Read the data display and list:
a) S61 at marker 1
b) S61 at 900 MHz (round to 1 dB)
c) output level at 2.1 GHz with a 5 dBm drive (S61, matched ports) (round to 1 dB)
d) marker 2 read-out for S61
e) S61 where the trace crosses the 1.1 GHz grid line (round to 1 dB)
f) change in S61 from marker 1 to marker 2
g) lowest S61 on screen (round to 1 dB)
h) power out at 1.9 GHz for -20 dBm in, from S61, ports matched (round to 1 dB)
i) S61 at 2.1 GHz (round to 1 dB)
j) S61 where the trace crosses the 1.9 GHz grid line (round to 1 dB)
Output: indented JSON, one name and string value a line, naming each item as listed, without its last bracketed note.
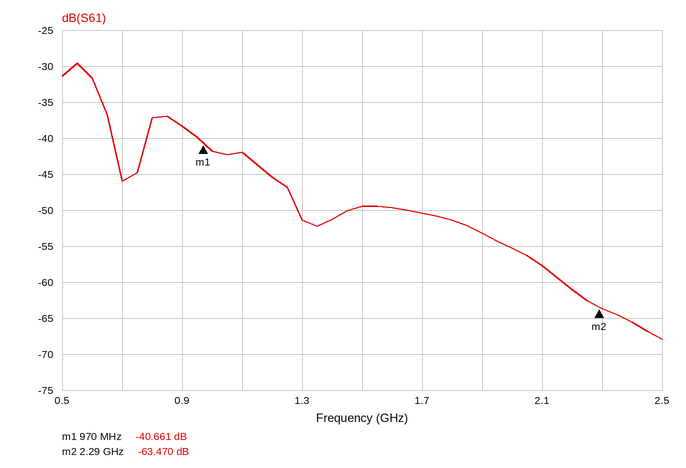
{
  "S61 at marker 1": "-40.661 dB",
  "S61 at 900 MHz": "-38 dB",
  "output level at 2.1 GHz with a 5 dBm drive (S61, matched ports)": "-53 dBm",
  "marker 2 read-out for S61": "-63.470 dB",
  "S61 where the trace crosses the 1.1 GHz grid line": "-42 dB",
  "change in S61 from marker 1 to marker 2": "-22.809 dB",
  "lowest S61 on screen": "-68 dB",
  "power out at 1.9 GHz for -20 dBm in, from S61, ports matched": "-73 dBm",
  "S61 at 2.1 GHz": "-58 dB",
  "S61 where the trace crosses the 1.9 GHz grid line": "-53 dB"
}
